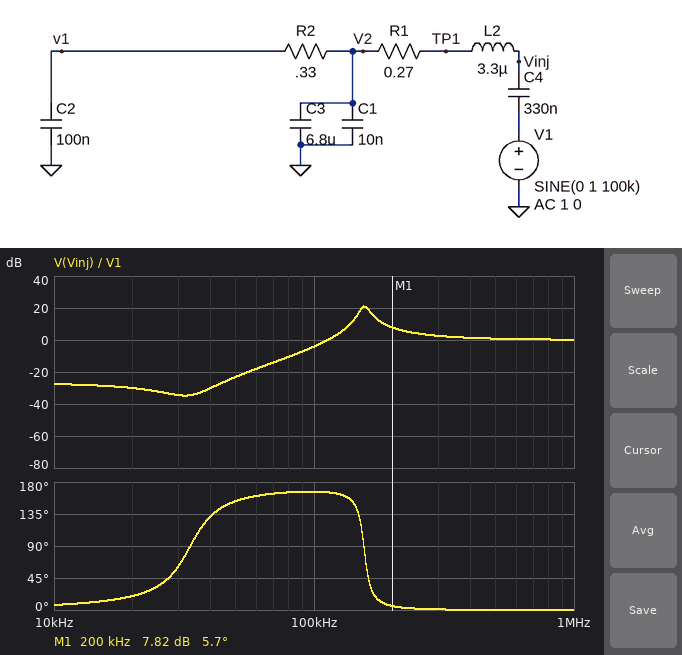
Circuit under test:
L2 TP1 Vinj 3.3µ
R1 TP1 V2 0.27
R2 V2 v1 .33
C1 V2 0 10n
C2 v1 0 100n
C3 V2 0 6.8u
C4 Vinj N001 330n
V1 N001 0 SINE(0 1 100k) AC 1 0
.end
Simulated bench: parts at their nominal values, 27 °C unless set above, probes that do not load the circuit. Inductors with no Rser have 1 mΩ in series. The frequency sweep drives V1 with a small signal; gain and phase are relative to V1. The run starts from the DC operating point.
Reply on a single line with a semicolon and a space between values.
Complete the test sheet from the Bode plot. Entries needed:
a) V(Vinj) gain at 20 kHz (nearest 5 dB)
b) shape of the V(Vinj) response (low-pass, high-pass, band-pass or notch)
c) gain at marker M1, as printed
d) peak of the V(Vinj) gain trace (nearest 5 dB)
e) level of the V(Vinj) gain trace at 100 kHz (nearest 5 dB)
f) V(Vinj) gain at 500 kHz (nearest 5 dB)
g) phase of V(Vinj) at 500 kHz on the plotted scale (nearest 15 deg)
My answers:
-30 dB; band-pass; 7.82 dB; 20 dB; -5 dB; 0 dB; 0 deg
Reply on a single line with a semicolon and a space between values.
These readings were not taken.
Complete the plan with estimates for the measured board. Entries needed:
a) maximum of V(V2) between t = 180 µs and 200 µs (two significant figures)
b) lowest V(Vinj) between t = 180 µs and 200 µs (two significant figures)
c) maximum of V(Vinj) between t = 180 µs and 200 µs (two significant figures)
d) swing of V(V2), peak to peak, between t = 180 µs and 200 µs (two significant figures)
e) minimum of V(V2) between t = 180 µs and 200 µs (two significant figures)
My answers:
77 mV; -620 mV; 620 mV; 150 mV; -77 mV
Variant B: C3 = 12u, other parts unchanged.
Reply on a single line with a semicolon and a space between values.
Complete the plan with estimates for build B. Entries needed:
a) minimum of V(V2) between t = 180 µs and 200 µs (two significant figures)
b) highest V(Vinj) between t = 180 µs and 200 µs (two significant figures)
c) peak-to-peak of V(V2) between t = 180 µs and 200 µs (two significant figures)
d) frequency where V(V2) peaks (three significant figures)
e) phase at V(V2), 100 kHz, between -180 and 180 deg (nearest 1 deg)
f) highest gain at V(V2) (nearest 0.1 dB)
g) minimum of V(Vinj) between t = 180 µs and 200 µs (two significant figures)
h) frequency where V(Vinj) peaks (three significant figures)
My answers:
-45 mV; 680 mV; 91 mV; 154 kHz; -5 deg; -10.1 dB; -680 mV; 155 kHz
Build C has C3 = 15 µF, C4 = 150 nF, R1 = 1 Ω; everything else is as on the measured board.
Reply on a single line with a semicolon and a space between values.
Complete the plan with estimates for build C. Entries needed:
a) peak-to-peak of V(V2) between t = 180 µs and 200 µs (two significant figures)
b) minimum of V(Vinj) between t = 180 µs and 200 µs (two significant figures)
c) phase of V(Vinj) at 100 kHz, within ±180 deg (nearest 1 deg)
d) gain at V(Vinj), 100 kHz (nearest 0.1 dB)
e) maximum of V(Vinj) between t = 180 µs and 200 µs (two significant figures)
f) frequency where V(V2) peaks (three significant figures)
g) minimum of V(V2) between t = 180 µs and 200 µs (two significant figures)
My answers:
24 mV; -250 mV; 146 deg; -11.9 dB; 250 mV; 225 kHz; -12 mV
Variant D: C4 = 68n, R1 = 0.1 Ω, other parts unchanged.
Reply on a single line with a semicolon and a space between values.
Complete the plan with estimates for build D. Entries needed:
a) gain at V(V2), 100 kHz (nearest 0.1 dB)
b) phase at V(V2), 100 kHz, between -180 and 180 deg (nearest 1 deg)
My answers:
-39.4 dB; 0 deg
